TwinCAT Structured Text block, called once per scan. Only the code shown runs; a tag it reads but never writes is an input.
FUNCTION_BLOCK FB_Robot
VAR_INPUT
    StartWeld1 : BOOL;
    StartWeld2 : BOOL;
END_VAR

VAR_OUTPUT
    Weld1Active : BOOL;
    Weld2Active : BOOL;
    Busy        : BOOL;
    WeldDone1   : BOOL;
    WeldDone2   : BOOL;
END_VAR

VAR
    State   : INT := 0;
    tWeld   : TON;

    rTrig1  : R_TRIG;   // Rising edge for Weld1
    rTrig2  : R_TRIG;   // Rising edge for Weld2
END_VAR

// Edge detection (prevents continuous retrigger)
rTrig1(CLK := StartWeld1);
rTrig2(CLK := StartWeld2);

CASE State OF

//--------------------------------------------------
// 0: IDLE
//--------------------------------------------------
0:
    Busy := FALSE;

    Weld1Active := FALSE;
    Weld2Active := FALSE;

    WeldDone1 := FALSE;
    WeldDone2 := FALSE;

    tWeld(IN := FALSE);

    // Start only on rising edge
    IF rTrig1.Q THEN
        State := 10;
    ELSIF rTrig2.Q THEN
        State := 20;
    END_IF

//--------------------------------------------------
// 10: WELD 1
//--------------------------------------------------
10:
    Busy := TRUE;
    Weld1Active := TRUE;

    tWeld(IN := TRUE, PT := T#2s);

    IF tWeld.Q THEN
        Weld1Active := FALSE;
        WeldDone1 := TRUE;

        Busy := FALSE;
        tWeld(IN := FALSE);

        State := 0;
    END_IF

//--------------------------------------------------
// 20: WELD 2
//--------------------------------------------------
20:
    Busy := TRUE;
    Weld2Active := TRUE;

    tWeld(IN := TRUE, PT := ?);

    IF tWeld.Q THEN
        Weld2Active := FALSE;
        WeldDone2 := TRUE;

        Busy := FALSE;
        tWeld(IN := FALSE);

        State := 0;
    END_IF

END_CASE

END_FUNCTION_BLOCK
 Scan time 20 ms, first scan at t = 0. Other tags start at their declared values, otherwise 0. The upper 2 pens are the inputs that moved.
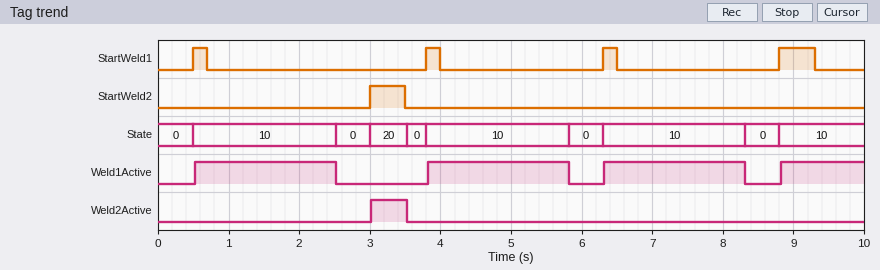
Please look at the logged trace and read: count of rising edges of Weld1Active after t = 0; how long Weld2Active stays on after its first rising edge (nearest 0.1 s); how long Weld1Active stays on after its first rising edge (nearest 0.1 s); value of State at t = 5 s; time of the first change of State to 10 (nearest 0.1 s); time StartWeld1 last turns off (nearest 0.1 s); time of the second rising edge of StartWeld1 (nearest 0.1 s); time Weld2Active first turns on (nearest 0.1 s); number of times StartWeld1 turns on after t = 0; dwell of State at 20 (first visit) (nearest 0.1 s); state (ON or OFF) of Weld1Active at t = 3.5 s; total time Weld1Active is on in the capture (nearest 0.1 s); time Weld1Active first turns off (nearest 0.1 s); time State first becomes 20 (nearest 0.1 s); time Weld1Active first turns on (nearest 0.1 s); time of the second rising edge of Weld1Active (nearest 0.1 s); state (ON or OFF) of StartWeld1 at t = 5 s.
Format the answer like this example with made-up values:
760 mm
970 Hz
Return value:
4
0.5 s
2.0 s
10
0.5 s
9.3 s
3.8 s
3.0 s
4
0.5 s
OFF
7.2 s
2.5 s
3.0 s
0.5 s
3.8 s
OFF
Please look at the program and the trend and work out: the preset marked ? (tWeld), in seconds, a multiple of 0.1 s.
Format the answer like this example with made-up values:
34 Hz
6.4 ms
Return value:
0.5 s
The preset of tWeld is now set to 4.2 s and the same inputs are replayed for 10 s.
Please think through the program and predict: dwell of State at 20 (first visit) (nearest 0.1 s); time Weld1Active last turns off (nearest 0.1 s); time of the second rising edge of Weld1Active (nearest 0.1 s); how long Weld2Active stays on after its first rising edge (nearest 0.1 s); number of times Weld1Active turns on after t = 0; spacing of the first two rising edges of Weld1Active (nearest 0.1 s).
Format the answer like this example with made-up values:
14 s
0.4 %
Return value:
4.2 s
2.5 s
8.8 s
4.2 s
2
8.3 s
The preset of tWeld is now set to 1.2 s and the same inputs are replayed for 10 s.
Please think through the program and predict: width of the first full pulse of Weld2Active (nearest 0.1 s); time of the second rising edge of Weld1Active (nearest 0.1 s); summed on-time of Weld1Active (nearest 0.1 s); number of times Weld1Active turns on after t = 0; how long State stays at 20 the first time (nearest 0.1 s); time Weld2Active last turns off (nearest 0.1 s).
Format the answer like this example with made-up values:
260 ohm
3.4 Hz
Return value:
1.2 s
6.3 s
5.2 s
3
1.2 s
4.2 s
